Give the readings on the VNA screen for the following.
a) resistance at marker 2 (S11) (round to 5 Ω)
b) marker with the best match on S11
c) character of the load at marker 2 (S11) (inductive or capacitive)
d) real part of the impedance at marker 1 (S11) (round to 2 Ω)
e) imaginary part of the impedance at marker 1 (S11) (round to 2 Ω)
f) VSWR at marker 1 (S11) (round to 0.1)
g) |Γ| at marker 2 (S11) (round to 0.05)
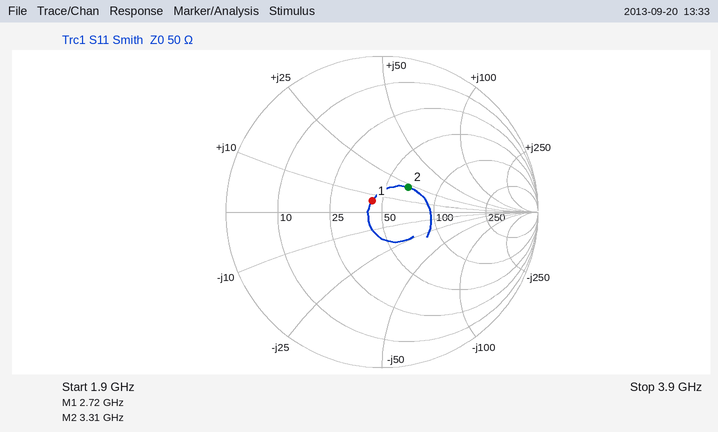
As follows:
65 Ω
marker 1
inductive
44 Ω
+6 Ω
1.2
0.25
